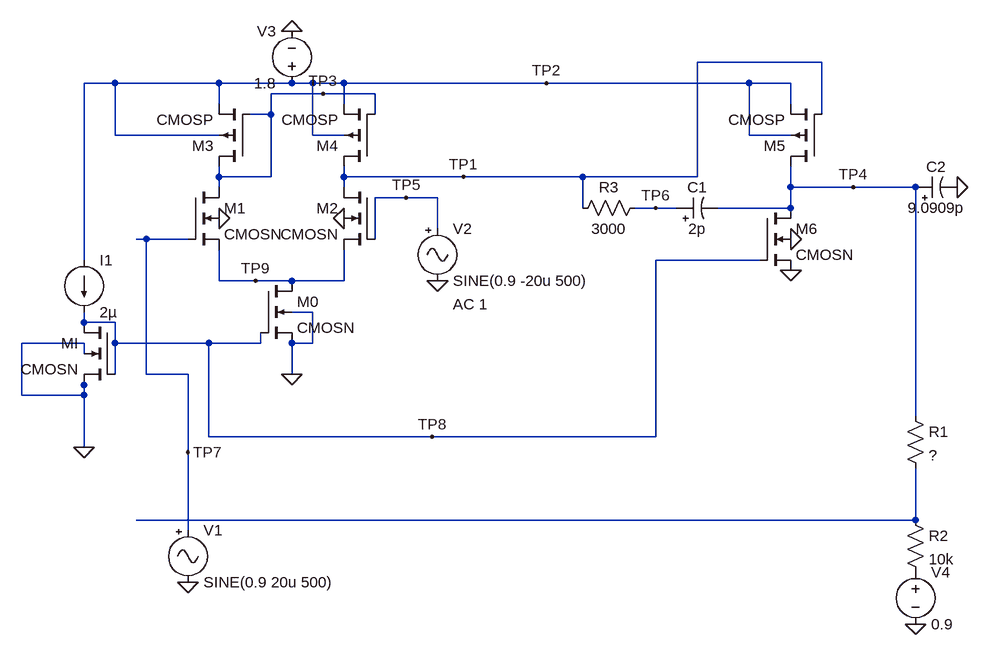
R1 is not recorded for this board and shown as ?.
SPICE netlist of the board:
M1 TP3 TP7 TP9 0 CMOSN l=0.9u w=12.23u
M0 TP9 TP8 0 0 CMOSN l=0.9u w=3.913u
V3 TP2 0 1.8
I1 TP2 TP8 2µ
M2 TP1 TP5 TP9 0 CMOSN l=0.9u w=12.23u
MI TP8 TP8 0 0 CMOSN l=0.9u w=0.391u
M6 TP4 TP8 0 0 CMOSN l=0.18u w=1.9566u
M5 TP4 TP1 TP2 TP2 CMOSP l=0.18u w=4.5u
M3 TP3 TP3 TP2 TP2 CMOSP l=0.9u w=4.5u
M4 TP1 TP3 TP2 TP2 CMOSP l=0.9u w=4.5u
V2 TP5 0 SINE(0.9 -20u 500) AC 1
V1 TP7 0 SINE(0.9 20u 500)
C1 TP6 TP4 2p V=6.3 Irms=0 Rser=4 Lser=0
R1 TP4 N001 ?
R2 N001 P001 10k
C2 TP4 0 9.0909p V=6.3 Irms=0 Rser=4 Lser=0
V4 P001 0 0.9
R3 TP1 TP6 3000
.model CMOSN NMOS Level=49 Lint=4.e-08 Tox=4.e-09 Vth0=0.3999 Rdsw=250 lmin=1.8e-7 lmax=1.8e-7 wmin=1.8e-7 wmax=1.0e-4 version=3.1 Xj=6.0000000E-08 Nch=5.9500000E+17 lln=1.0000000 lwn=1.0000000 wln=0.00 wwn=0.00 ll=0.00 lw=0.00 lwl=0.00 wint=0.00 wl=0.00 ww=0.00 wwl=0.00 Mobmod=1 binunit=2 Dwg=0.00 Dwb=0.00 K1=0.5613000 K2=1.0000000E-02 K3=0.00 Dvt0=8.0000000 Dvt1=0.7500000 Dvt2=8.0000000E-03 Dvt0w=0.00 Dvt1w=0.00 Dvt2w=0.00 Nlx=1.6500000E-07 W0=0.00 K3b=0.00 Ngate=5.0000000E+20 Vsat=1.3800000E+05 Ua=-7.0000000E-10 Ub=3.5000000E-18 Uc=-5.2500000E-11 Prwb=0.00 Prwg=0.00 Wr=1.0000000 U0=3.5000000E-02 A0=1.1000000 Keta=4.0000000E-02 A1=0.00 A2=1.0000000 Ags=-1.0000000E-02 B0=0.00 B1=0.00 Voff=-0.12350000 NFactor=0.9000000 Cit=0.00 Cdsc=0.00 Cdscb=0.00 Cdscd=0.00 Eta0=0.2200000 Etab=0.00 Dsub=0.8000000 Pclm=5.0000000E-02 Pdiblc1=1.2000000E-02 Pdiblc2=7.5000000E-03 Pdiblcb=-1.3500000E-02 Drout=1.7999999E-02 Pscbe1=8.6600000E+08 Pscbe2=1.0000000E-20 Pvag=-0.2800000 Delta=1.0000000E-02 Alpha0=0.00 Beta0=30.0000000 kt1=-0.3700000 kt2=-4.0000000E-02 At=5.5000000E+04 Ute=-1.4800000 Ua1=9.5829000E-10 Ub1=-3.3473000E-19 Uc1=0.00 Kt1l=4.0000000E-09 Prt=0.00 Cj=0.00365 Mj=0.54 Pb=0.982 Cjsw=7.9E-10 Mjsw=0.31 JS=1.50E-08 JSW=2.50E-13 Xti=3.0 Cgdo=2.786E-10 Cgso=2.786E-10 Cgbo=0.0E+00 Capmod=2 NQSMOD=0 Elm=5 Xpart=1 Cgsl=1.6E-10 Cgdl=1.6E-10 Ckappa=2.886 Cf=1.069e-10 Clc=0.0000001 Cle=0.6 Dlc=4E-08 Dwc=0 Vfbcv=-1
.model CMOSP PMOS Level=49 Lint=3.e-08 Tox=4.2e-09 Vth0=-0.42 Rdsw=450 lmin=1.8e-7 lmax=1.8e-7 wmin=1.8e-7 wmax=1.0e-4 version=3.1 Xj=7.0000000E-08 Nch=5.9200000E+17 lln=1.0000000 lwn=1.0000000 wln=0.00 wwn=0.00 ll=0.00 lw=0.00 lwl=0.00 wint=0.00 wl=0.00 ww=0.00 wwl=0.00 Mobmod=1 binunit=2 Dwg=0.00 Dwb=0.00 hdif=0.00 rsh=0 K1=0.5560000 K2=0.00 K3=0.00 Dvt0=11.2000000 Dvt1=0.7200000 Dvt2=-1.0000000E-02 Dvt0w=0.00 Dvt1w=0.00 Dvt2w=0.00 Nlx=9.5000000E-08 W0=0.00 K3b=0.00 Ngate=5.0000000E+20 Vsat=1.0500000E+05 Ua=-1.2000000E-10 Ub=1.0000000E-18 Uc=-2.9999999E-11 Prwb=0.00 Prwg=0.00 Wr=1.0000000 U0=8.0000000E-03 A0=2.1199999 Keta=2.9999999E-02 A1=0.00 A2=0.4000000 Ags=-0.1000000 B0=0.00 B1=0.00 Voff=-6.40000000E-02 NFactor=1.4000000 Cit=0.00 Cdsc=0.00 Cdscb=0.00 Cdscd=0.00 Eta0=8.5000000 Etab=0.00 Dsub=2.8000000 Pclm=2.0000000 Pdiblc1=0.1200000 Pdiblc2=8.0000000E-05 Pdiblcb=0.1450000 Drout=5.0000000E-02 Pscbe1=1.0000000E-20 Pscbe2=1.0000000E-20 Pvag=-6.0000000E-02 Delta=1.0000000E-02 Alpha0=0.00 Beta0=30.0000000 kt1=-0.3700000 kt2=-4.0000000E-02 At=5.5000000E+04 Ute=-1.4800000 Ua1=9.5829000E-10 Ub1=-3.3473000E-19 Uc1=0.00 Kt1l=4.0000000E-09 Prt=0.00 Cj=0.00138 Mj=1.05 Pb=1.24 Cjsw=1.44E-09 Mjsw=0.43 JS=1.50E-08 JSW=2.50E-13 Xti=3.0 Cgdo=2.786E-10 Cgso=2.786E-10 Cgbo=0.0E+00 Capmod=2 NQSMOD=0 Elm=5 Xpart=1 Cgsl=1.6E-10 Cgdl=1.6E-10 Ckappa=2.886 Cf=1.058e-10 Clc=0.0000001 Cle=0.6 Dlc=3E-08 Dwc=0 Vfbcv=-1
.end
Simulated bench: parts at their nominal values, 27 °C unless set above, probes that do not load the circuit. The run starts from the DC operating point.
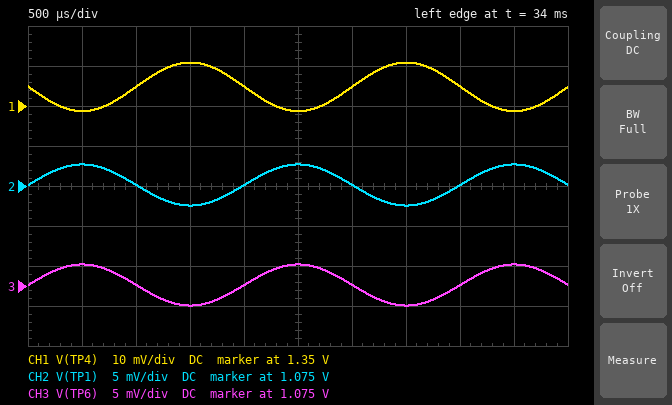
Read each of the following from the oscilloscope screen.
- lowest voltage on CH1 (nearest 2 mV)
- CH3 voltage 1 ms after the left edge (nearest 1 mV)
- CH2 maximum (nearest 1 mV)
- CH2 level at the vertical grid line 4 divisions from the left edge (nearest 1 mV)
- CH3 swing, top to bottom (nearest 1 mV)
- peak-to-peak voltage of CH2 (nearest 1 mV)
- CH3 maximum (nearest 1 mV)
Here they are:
1.348 V
1.075 V
1.078 V
1.075 V
5 mV
5 mV
1.078 V
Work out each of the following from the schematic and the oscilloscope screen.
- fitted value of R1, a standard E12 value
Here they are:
8.2 kΩ
